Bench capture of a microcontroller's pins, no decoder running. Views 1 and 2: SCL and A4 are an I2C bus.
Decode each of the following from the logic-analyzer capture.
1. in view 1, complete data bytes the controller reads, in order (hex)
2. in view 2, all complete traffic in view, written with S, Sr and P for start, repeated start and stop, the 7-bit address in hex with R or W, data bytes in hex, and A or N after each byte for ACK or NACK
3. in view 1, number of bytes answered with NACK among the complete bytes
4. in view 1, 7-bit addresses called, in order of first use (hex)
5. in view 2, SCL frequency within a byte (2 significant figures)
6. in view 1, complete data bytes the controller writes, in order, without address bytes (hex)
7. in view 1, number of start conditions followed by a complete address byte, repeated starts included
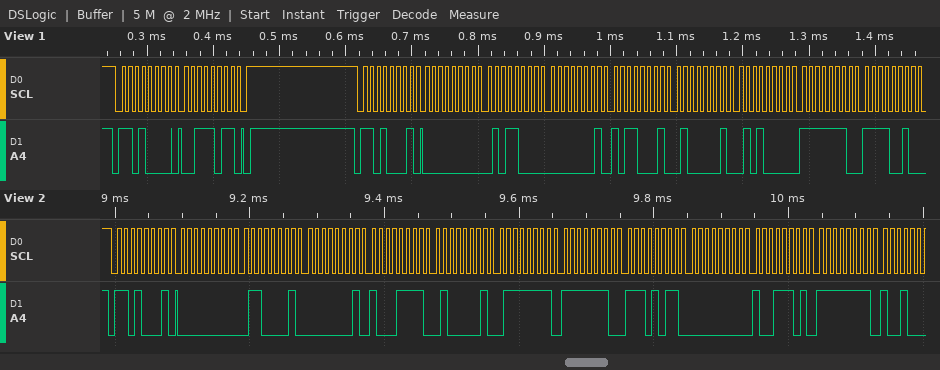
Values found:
00 58 01 B1 41 50 FE F2
S 68R A 00 A 61 A 01 A 8F A 41 A 7F A FE A EB A 00 A 9D A FF A
0
0x68
100 kHz
3B
2
